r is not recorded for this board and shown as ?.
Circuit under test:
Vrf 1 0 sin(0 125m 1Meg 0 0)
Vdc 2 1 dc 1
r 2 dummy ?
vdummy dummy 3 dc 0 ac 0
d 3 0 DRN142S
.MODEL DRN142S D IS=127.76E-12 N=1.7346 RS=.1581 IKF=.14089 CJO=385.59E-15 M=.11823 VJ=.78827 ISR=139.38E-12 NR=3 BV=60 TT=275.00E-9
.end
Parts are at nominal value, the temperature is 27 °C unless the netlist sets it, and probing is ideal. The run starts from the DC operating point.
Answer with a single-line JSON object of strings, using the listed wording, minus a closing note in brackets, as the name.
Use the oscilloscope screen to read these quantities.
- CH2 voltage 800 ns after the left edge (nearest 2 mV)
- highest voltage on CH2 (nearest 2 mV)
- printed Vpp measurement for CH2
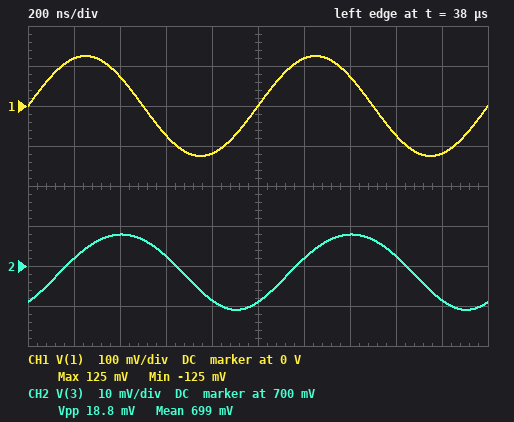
{"CH2 voltage 800 ns after the left edge": "692 mV", "highest voltage on CH2": "708 mV", "printed Vpp measurement for CH2": "18.8 mV"}
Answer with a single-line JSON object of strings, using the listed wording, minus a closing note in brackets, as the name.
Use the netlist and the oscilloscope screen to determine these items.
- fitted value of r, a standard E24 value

{"fitted value of r, a standard E24 value": "430 Ω"}
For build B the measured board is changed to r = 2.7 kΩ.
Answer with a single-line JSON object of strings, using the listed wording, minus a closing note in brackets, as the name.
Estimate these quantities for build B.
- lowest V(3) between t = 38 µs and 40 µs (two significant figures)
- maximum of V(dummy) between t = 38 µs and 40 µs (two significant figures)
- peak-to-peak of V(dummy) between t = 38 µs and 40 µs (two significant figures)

{"lowest V(3) between t = 38 µs and 40 µs": "620 mV", "maximum of V(dummy) between t = 38 µs and 40 µs": "630 mV", "peak-to-peak of V(dummy) between t = 38 µs and 40 µs": "15 mV"}
